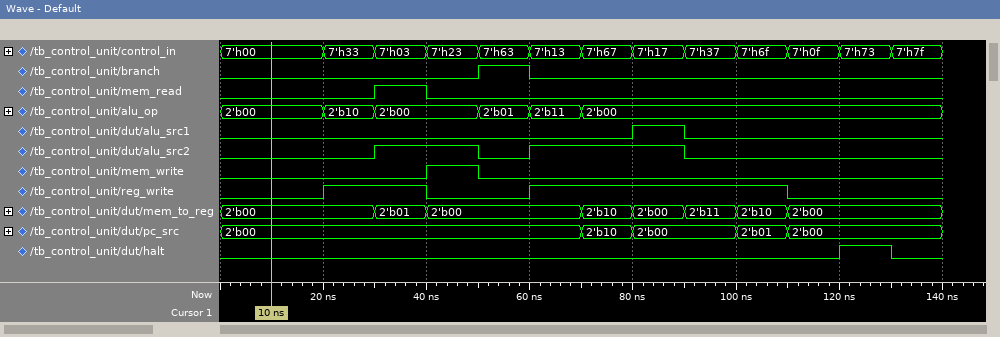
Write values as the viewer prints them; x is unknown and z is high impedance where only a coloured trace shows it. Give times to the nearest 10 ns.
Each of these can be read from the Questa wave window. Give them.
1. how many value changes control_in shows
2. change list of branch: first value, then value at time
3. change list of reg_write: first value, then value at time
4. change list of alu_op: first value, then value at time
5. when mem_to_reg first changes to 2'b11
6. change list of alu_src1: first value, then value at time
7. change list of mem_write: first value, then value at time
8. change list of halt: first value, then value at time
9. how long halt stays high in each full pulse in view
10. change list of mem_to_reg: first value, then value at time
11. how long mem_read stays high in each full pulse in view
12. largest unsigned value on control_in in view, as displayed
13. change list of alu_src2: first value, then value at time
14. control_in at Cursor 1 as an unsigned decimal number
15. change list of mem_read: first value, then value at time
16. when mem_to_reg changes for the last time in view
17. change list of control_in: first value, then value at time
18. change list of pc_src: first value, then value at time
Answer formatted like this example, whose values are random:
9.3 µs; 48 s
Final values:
12; 0, 1 at 50 ns, 0 at 60 ns; 0, 1 at 20 ns, 0 at 40 ns, 1 at 60 ns, 0 at 110 ns; 2'b00, 2'b10 at 20 ns, 2'b00 at 30 ns, 2'b01 at 50 ns, 2'b11 at 60 ns, 2'b00 at 70 ns; 90 ns; 0, 1 at 80 ns, 0 at 90 ns; 0, 1 at 40 ns, 0 at 50 ns; 0, 1 at 120 ns, 0 at 130 ns; 10 ns; 2'b00, 2'b01 at 30 ns, 2'b00 at 40 ns, 2'b10 at 70 ns, 2'b00 at 80 ns, 2'b11 at 90 ns, 2'b10 at 100 ns, 2'b00 at 110 ns; 10 ns; 7'h7f; 0, 1 at 30 ns, 0 at 50 ns, 1 at 60 ns, 0 at 90 ns; 0; 0, 1 at 30 ns, 0 at 40 ns; 110 ns; 7'h00, 7'h33 at 20 ns, 7'h03 at 30 ns, 7'h23 at 40 ns, 7'h63 at 50 ns, 7'h13 at 60 ns, 7'h67 at 70 ns, 7'h17 at 80 ns, 7'h37 at 90 ns, 7'h6f at 100 ns, 7'h0f at 110 ns, 7'h73 at 120 ns, 7'h7f at 130 ns; 2'b00, 2'b10 at 70 ns, 2'b00 at 80 ns, 2'b01 at 100 ns, 2'b00 at 110 ns
